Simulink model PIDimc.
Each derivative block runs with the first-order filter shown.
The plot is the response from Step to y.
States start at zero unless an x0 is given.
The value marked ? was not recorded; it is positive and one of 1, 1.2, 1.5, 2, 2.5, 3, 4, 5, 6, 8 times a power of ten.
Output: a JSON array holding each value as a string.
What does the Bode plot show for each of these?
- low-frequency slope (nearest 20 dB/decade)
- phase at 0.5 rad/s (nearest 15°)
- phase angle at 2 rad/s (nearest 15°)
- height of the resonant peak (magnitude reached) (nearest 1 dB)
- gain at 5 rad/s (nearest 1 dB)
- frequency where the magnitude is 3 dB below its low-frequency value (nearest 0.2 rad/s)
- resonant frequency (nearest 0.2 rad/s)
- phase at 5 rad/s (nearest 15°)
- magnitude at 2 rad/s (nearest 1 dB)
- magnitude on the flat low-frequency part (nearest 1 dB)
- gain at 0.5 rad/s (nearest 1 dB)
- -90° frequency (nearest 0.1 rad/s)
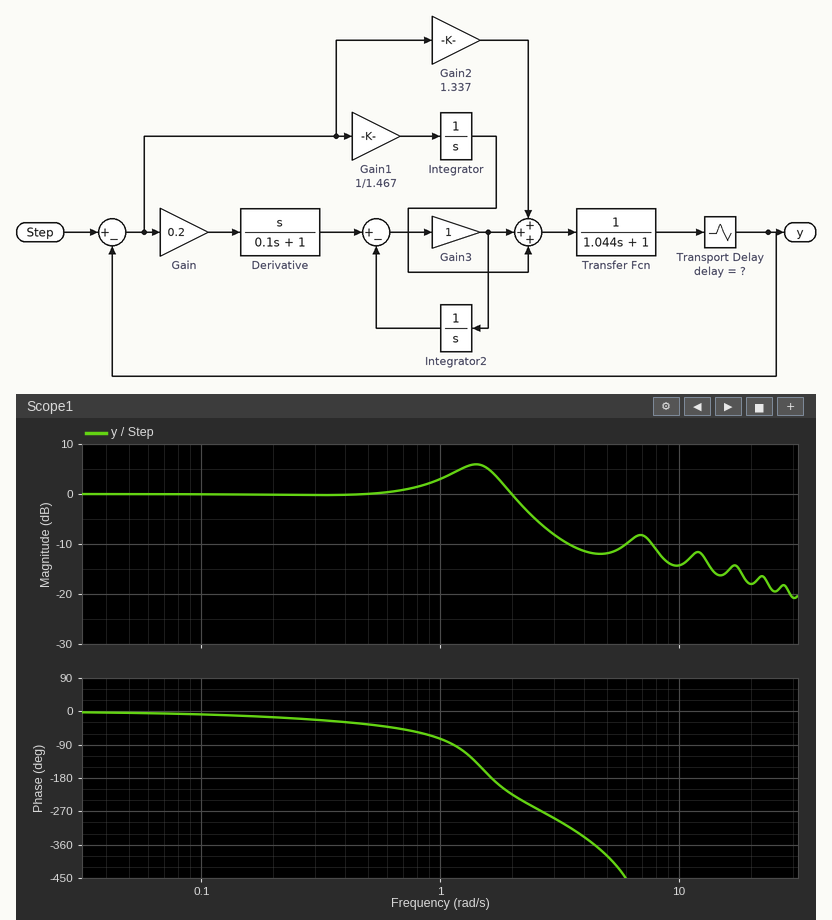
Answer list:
["0 dB/decade", "-30°", "-225°", "6 dB", "-12 dB", "2.2 rad/s", "1.4 rad/s", "-390°", "0 dB", "0 dB", "0 dB", "1.1 rad/s"]
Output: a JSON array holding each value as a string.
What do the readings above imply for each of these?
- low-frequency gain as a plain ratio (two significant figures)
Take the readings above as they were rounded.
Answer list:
["1.0"]
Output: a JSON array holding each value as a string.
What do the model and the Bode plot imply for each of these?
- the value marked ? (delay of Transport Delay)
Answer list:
["1.2"]
